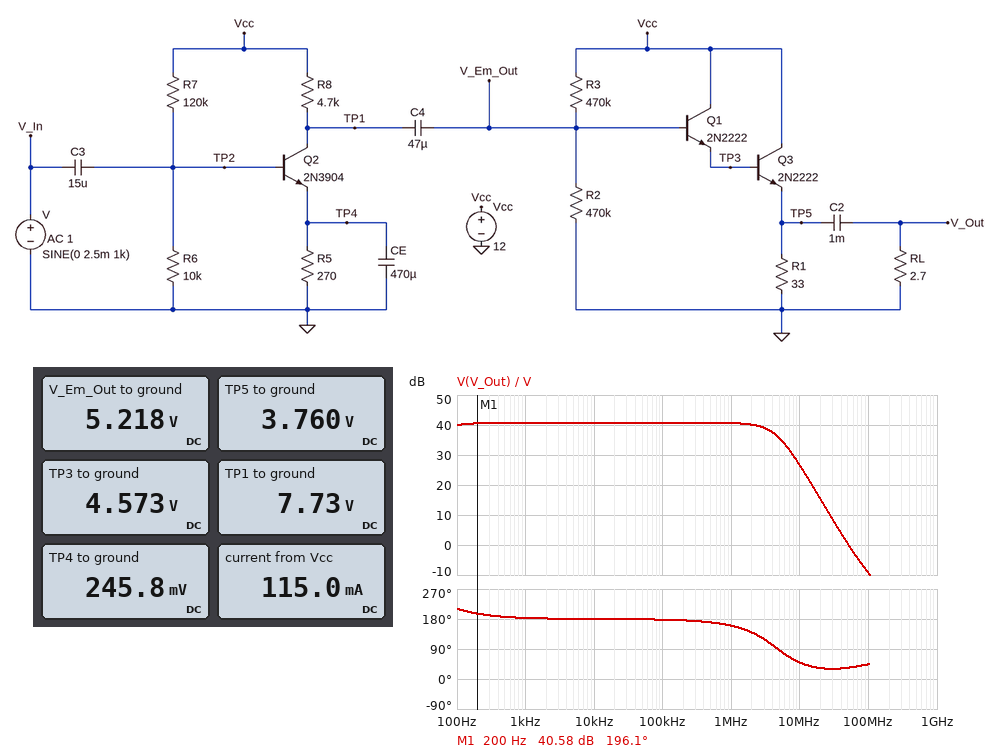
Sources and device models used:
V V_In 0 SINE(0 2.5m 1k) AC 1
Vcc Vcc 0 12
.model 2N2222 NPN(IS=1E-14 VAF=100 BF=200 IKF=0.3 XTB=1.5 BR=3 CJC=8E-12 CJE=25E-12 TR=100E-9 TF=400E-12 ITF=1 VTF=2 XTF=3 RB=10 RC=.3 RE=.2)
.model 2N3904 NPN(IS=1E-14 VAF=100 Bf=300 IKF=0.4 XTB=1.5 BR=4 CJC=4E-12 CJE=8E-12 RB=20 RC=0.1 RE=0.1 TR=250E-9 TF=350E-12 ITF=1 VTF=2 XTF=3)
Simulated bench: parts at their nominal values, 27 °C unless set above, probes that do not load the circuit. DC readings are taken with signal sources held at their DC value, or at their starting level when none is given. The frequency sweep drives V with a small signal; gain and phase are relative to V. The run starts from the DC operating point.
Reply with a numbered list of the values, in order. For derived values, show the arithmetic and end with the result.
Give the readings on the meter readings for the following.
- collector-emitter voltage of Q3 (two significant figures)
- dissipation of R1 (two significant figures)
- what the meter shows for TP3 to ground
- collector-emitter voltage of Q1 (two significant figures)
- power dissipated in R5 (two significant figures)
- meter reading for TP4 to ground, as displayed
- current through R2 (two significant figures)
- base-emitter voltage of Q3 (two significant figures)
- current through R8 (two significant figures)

1. 12 V - 3.76 V = 8.2 V
2. (3.76 V)^2 / 33 Ω = 430 mW
3. 4.573 V
4. 12 V - 4.573 V = 7.4 V
5. (245.8 mV)^2 / 270 Ω = 220 µW
6. 245.8 mV
7. (5.218 V) / 470 kΩ = 11 µA
8. 4.573 V - 3.76 V = 810 mV
9. (12 V - 7.73 V) / 4.7 kΩ = 910 µA
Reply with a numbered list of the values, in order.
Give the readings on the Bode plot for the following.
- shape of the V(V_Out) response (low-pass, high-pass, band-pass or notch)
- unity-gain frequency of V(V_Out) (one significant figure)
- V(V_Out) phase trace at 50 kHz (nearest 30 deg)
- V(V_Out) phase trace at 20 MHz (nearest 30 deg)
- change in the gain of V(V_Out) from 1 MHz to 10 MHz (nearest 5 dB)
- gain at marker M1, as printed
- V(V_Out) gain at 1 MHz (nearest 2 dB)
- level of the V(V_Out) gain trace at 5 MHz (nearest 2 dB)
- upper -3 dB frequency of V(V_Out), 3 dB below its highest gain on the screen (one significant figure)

1. low-pass
2. 50 MHz
3. 180 deg
4. 30 deg
5. -15 dB
6. 40.58 dB
7. 40 dB
8. 36 dB
9. 4 MHz
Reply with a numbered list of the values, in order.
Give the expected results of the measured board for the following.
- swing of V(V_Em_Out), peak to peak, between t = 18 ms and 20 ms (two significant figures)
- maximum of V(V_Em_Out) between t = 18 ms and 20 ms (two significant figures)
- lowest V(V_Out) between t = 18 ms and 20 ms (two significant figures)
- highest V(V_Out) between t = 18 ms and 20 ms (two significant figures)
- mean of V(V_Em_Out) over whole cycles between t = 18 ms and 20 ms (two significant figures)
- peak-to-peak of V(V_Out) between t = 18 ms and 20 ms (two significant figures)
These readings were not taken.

1. 740 mV
2. 5.6 V
3. -250 mV
4. 260 mV
5. 5.2 V
6. 510 mV
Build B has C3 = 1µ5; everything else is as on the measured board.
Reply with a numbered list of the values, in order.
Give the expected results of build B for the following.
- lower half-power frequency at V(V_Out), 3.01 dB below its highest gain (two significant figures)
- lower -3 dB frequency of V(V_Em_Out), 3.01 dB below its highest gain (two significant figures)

1. 58 Hz
2. 30 Hz
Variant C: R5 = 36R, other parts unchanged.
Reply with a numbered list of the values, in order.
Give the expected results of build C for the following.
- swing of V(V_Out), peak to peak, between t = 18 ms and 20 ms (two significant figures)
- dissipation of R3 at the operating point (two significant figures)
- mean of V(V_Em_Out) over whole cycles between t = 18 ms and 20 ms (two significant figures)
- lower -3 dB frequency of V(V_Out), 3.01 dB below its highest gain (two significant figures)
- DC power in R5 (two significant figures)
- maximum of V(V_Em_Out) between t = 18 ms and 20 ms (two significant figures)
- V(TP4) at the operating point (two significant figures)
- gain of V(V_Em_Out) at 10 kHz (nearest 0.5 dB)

1. 750 mV
2. 98 µW
3. 5.5 V
4. 160 Hz
5. 230 µW
6. 6.2 V
7. 91 mV
8. 32.0 dB
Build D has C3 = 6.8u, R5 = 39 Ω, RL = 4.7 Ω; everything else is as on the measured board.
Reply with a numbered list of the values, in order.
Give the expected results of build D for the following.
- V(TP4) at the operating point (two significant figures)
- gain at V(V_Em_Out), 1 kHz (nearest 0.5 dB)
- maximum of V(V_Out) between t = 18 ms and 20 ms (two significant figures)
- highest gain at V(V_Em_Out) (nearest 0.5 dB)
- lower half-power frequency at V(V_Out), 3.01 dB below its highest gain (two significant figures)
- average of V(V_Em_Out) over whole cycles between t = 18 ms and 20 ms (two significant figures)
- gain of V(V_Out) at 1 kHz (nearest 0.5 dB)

1. 98 mV
2. 32.5 dB
3. 590 mV
4. 33.0 dB
5. 310 Hz
6. 5.6 V
7. 31.0 dB
